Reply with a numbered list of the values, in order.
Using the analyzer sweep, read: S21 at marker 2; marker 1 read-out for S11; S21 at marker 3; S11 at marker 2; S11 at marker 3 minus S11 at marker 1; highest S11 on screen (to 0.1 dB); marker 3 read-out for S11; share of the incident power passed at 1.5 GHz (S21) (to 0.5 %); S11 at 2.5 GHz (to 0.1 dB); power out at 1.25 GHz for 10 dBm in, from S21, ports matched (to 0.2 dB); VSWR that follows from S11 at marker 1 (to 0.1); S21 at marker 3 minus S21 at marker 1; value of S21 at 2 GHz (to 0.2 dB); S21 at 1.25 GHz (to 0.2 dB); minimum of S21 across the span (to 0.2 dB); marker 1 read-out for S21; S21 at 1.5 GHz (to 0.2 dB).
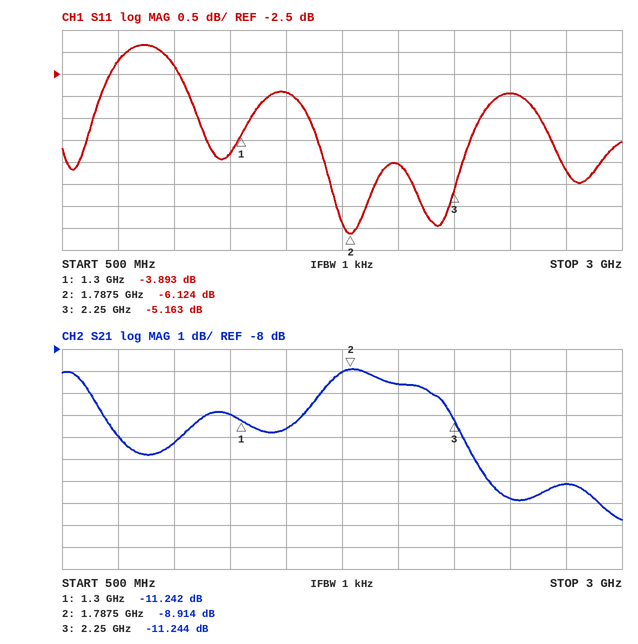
1. -8.914 dB
2. -3.893 dB
3. -11.244 dB
4. -6.124 dB
5. -1.270 dB
6. -1.8 dB
7. -5.163 dB
8. 7.0 %
9. -2.9 dB
10. -1.0 dBm
11. 4.5
12. -0.002 dB
13. -9.6 dB
14. -11.0 dB
15. -15.8 dB
16. -11.242 dB
17. -11.6 dB
